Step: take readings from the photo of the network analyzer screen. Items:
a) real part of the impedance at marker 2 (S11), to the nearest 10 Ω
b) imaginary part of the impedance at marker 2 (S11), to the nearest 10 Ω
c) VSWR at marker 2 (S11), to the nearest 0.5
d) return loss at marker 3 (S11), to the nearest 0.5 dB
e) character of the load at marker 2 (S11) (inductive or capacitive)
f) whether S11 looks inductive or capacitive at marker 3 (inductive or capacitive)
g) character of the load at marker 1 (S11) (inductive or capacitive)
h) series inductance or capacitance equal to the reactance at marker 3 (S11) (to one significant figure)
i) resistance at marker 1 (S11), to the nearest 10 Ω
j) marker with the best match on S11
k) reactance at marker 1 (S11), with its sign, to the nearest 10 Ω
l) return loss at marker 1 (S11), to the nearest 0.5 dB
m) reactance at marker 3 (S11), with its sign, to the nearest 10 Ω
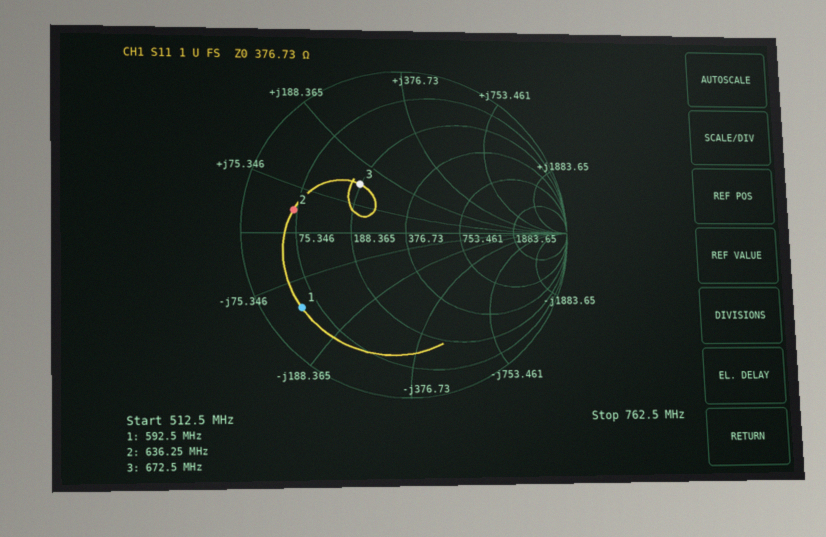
70 Ω
+40 Ω
5.5
8.0 dB
inductive
inductive
capacitive
30 nH
50 Ω
marker 3
-120 Ω
2.0 dB
+130 Ω
